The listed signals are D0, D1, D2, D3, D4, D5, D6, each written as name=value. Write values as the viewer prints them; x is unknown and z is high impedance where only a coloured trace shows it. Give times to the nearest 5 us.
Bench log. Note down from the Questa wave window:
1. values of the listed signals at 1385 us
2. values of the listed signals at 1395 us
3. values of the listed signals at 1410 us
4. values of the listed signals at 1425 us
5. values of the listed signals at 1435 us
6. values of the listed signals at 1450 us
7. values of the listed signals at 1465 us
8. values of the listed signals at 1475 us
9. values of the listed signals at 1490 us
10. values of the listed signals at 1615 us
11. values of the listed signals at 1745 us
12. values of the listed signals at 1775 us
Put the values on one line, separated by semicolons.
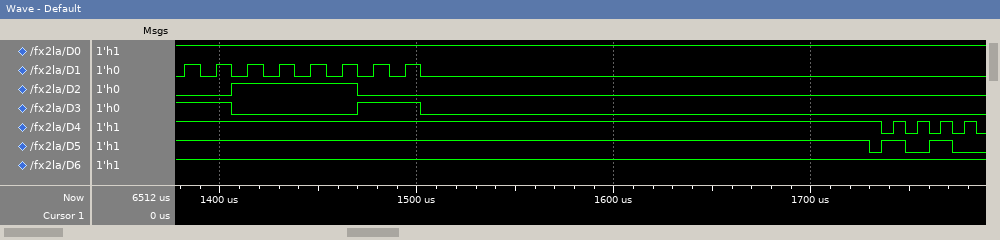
D0=1, D1=1, D2=0, D3=1, D4=1, D5=1, D6=1; D0=1, D1=0, D2=0, D3=1, D4=1, D5=1, D6=1; D0=1, D1=0, D2=1, D3=0, D4=1, D5=1, D6=1; D0=1, D1=0, D2=1, D3=0, D4=1, D5=1, D6=1; D0=1, D1=1, D2=1, D3=0, D4=1, D5=1, D6=1; D0=1, D1=1, D2=1, D3=0, D4=1, D5=1, D6=1; D0=1, D1=1, D2=1, D3=0, D4=1, D5=1, D6=1; D0=1, D1=0, D2=0, D3=1, D4=1, D5=1, D6=1; D0=1, D1=0, D2=0, D3=1, D4=1, D5=1, D6=1; D0=1, D1=0, D2=0, D3=0, D4=1, D5=1, D6=1; D0=1, D1=0, D2=0, D3=0, D4=1, D5=1, D6=1; D0=1, D1=0, D2=0, D3=0, D4=0, D5=0, D6=1
